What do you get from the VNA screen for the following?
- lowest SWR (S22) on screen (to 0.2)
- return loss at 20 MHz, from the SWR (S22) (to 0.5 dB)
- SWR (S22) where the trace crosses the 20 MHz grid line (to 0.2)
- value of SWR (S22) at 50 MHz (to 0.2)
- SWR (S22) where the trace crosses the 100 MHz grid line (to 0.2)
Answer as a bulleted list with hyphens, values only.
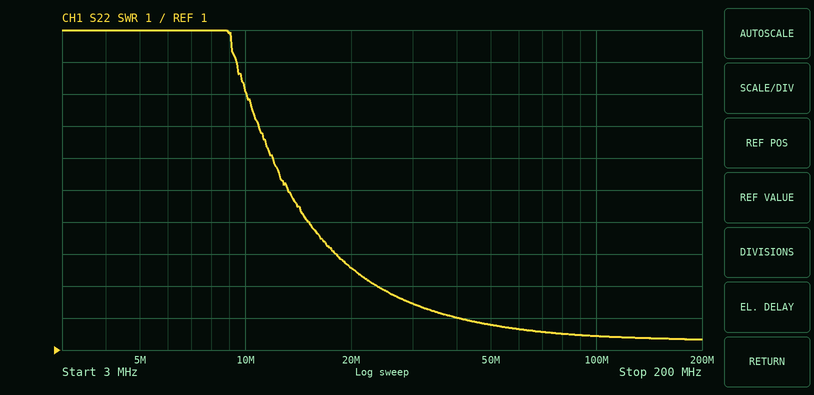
- 1.4
- 5.0 dB
- 3.6
- 1.8
- 1.4
